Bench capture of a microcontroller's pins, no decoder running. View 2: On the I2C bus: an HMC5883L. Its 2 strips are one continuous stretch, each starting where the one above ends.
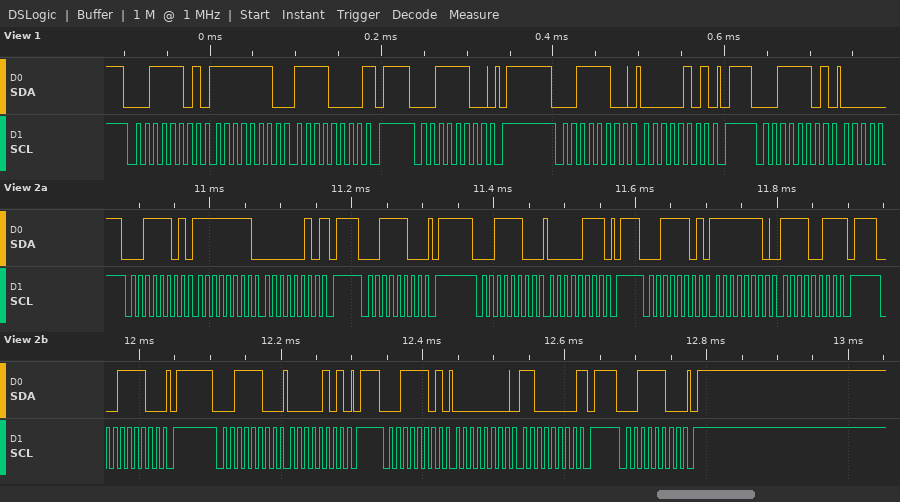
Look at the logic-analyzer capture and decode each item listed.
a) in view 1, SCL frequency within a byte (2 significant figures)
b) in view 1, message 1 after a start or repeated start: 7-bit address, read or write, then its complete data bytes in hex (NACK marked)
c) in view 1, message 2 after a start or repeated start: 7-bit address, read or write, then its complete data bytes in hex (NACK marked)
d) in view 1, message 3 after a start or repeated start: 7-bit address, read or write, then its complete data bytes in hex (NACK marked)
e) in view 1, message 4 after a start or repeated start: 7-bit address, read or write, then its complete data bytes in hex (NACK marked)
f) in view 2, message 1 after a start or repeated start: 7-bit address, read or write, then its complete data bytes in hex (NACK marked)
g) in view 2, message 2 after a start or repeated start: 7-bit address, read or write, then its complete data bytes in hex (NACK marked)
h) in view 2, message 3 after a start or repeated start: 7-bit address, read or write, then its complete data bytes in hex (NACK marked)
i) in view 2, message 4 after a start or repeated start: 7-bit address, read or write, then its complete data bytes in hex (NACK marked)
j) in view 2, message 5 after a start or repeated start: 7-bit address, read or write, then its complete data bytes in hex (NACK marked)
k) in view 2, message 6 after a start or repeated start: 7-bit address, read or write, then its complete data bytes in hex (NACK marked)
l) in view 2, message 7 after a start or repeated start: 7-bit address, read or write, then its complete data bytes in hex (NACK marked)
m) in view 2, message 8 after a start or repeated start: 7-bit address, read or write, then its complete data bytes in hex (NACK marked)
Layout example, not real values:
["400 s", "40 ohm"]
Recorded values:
["100 kHz", "0x1E read: FE F0 NACK", "0x1E write", "0x1E write: 05", "0x1E read", "0x1E read: FF 02 NACK", "0x1E write", "0x1E write: 07", "0x1E read: FE F3 NACK", "0x1E write", "0x1E write: 05", "0x1E read: 00 C0 NACK", "0x1E write"]
